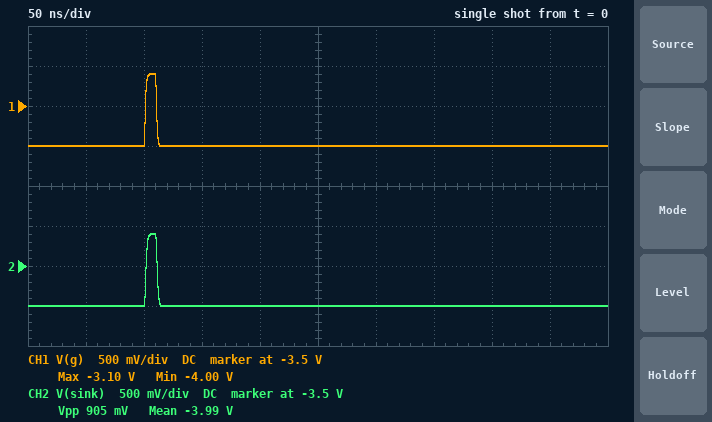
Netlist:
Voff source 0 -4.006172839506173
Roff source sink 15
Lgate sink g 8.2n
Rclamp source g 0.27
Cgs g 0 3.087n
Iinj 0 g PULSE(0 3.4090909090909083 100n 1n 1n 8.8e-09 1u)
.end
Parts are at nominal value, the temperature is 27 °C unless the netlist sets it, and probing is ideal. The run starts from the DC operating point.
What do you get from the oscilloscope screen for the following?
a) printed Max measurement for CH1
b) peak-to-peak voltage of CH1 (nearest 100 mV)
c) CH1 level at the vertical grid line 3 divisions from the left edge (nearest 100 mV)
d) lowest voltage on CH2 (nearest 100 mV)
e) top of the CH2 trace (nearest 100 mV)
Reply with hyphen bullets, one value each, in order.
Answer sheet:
- -3.10 V
- 900 mV
- -4.0 V
- -4.0 V
- -3.1 V
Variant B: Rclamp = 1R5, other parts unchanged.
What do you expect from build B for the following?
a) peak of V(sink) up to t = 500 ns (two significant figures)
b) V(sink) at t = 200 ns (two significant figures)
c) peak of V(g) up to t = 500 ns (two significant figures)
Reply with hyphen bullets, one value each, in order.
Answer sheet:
- 100 mV
- -4.0 V
- 150 mV
